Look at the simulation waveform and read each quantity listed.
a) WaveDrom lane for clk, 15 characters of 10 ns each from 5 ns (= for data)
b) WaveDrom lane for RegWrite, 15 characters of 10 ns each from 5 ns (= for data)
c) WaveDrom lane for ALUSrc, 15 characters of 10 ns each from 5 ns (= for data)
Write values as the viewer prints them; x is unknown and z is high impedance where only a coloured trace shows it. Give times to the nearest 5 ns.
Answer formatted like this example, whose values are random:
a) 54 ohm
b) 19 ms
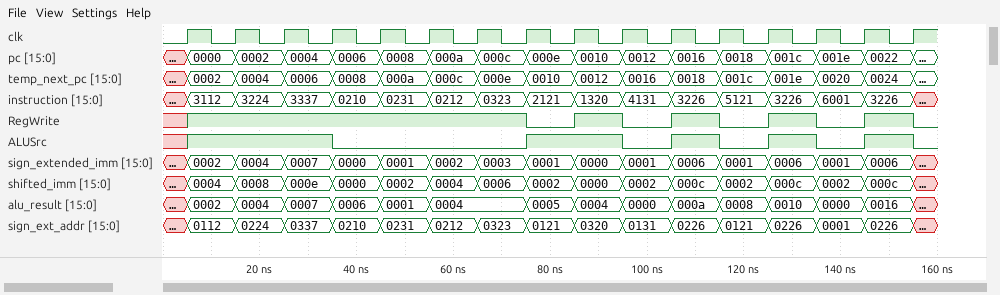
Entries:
a) {name: 'clk', wave: 'p..............'}
b) {name: 'RegWrite', wave: '1......01010101'}
c) {name: 'ALUSrc', wave: '1..0...1.010101'}
